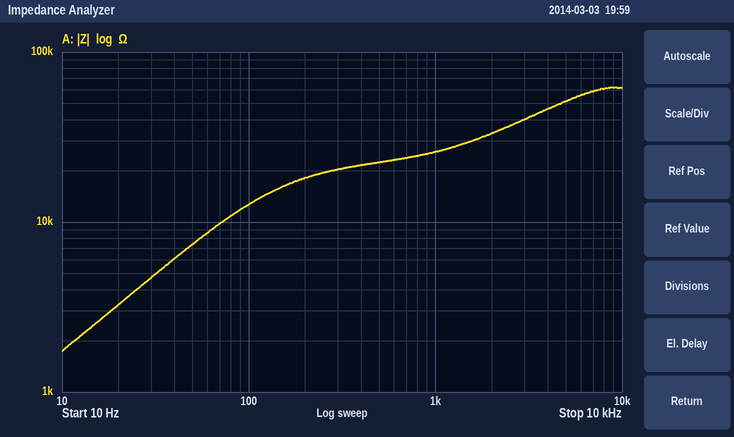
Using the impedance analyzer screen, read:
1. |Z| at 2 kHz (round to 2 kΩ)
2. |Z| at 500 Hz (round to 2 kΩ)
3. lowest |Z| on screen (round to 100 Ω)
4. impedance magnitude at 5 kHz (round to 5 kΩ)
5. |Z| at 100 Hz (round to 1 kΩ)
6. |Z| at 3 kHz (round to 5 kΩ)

34 kΩ
22 kΩ
1.7 kΩ
50 kΩ
13 kΩ
40 kΩ
